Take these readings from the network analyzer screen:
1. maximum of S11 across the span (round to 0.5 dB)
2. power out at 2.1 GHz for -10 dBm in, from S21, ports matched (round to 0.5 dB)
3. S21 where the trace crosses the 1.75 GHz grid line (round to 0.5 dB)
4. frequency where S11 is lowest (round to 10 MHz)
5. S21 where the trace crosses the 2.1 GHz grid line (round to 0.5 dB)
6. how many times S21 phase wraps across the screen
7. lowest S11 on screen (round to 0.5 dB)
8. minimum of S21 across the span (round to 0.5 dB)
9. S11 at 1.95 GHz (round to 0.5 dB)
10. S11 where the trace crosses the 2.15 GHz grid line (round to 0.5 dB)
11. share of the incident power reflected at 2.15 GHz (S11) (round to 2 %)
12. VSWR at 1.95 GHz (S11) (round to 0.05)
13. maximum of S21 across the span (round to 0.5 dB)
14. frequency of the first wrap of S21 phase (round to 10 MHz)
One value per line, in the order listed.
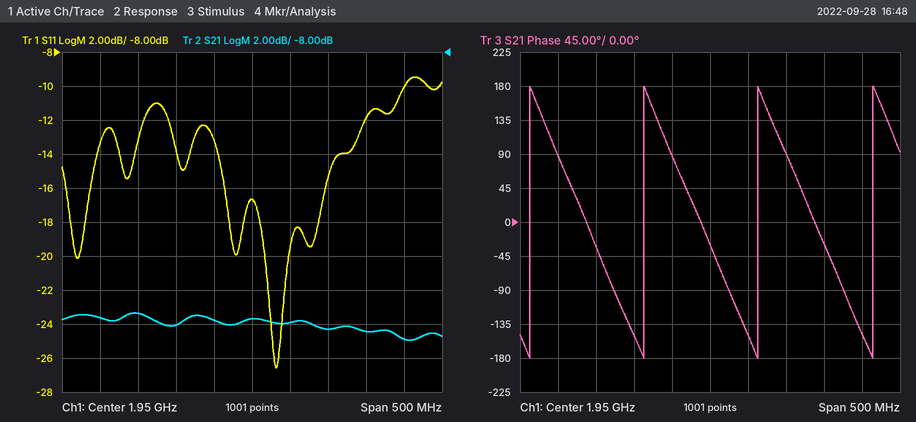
-9.5 dB
-34.5 dBm
-23.5 dB
1.98 GHz
-24.5 dB
4
-26.5 dB
-25.0 dB
-16.5 dB
-10.0 dB
10 %
1.35
-23.5 dB
1.71 GHz
